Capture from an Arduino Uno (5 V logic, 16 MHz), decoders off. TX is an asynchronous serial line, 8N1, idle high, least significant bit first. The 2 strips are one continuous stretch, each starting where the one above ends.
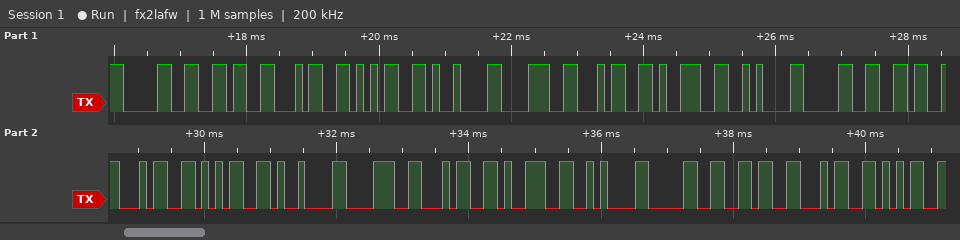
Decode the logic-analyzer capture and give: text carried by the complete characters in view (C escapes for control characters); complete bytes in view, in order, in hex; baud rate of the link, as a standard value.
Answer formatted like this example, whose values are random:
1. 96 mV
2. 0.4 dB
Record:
1. "0645\t849\n0645\t849\n0645"
2. 0x30 0x36 0x34 0x35 0x09 0x38 0x34 0x39 0x0A 0x30 0x36 0x34 0x35 0x09 0x38 0x34 0x39 0x0A 0x30 0x36 0x34 0x35
3. 9600 baud
